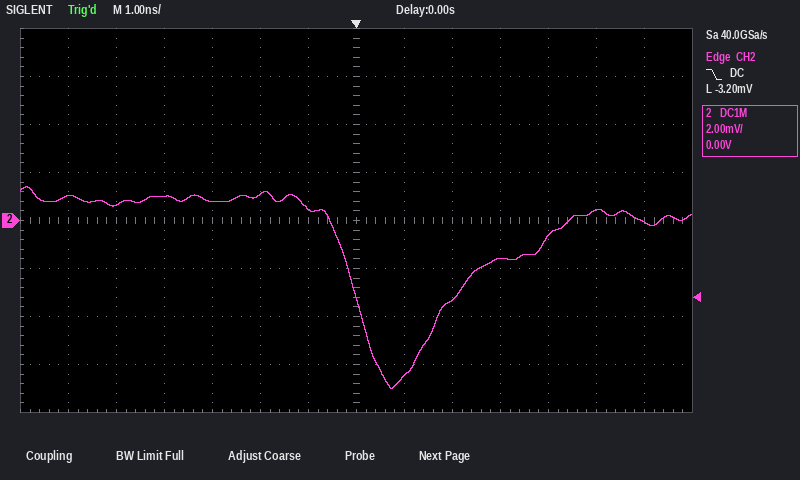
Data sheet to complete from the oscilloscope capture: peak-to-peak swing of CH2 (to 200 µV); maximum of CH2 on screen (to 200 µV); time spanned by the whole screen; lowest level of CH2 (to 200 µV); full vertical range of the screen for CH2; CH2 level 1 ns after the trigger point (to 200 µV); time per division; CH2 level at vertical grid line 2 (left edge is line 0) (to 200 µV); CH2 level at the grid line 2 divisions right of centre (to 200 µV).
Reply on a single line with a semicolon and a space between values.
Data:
8.4 mV; 1.4 mV; 14 ns; -7.0 mV; 16 mV; -6.4 mV; 1 ns; 600 µV; -3.4 mV
